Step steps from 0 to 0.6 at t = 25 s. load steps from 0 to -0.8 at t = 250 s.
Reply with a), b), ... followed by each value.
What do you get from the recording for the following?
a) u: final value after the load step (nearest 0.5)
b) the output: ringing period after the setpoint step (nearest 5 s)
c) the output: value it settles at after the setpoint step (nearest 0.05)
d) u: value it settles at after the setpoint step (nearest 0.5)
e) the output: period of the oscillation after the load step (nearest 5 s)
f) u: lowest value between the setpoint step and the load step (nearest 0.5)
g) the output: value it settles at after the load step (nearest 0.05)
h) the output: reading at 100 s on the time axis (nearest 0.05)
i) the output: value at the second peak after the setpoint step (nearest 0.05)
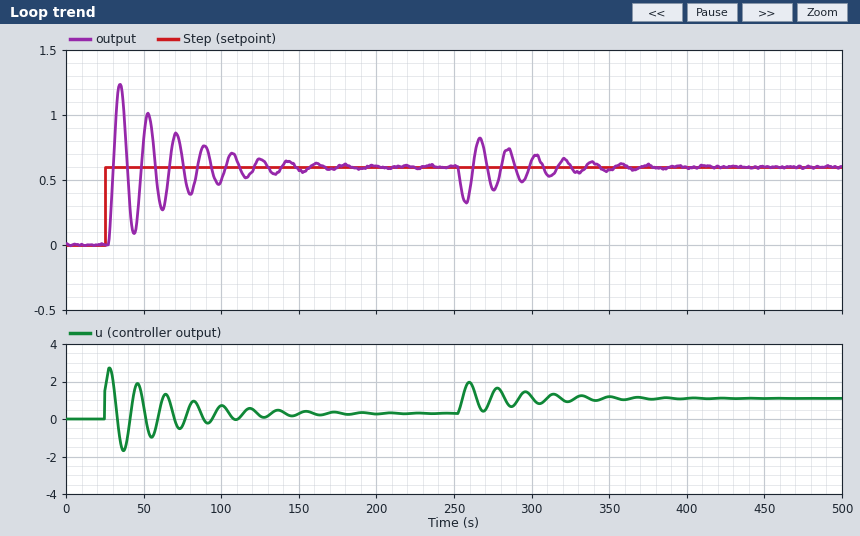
a) 1.0
b) 20 s
c) 0.60
d) 0.5
e) 20 s
f) -1.5
g) 0.60
h) 0.50
i) 1.00
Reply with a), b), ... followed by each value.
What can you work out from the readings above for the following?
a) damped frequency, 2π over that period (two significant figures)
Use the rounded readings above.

a) 0.31 rad/s
